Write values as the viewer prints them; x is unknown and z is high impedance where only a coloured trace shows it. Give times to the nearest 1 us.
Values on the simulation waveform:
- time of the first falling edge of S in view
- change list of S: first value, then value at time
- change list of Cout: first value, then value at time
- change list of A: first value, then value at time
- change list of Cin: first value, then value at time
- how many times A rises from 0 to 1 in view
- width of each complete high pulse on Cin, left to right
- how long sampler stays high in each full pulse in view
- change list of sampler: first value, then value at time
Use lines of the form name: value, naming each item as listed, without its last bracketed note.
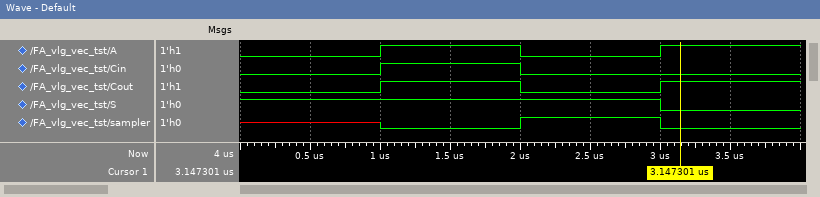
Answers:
time of the first falling edge of S in view: 3 us
change list of S: first value, then value at time: 1, 0 at 3 us
change list of Cout: first value, then value at time: 0, 1 at 1 us, 0 at 2 us, 1 at 3 us
change list of A: first value, then value at time: 0, 1 at 1 us, 0 at 2 us, 1 at 3 us
change list of Cin: first value, then value at time: 0, 1 at 1 us, 0 at 2 us
how many times A rises from 0 to 1 in view: 2
width of each complete high pulse on Cin, left to right: 1 us
how long sampler stays high in each full pulse in view: 1 us
change list of sampler: first value, then value at time: x, 0 at 1 us, 1 at 2 us, 0 at 3 us
